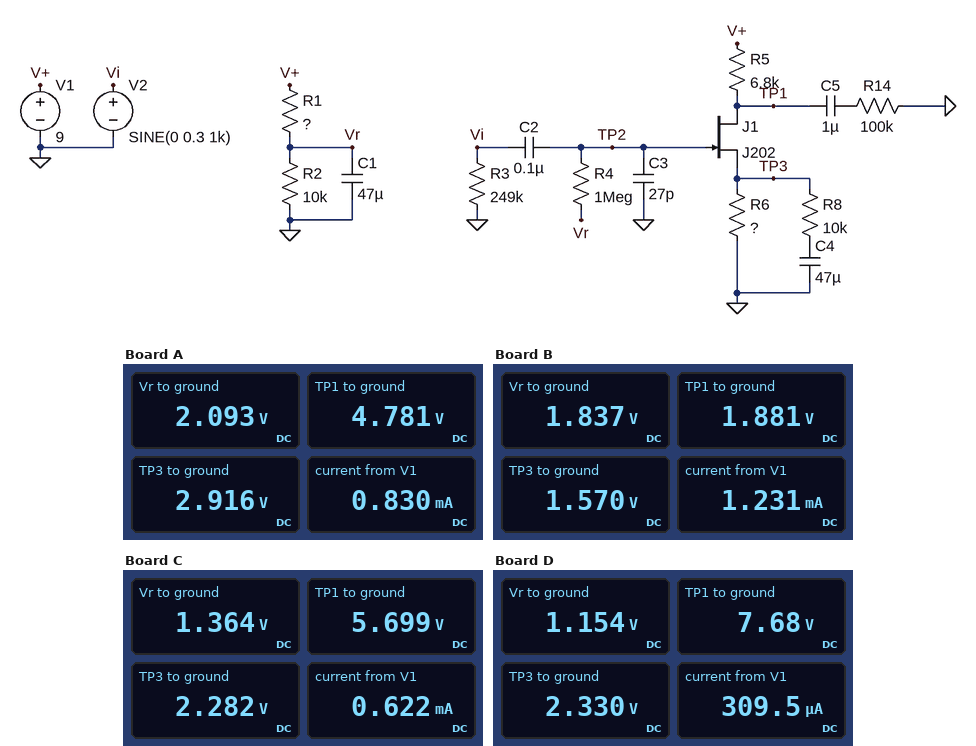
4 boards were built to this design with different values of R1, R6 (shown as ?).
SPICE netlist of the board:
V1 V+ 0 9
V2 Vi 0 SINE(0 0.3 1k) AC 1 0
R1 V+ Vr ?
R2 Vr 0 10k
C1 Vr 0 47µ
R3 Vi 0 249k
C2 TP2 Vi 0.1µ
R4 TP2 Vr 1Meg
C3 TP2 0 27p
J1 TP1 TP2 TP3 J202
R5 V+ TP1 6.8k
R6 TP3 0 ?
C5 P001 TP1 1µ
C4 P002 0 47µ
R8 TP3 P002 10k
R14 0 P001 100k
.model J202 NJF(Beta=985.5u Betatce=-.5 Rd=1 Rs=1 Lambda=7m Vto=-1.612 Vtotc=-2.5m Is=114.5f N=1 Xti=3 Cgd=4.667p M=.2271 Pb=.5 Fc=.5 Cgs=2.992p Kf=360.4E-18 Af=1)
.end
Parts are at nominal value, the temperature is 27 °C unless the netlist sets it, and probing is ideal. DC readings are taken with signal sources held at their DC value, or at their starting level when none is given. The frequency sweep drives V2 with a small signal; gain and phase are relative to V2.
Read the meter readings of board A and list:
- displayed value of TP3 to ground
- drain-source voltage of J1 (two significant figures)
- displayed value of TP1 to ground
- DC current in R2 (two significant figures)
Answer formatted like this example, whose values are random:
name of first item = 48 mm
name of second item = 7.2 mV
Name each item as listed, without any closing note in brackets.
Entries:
displayed value of TP3 to ground = 2.916 V
drain-source voltage of J1 = 1.9 V
displayed value of TP1 to ground = 4.781 V
DC current in R2 = 210 µA
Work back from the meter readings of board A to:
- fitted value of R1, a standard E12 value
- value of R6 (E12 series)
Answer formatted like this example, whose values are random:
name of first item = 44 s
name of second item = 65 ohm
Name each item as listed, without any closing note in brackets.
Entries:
fitted value of R1, a standard E12 value = 33 kΩ
value of R6 = 4.7 kΩ
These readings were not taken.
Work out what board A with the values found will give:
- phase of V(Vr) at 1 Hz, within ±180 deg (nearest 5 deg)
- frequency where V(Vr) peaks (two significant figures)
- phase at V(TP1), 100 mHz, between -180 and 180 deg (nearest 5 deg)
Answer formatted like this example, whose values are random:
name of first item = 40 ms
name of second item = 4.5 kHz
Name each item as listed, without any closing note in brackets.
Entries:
phase of V(Vr) at 1 Hz, within ±180 deg = -10 deg
frequency where V(Vr) peaks = 840 mHz
phase at V(TP1), 100 mHz, between -180 and 180 deg = -90 deg
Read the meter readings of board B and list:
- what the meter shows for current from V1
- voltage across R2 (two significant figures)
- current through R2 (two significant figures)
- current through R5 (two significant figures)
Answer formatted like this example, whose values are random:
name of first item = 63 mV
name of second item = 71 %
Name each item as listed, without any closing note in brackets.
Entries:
what the meter shows for current from V1 = 1.231 mA
voltage across R2 = 1.8 V
current through R2 = 180 µA
current through R5 = 1.0 mA
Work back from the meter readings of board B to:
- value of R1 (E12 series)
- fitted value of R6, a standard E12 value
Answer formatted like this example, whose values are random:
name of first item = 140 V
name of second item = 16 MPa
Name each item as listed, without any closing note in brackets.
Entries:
value of R1 = 39 kΩ
fitted value of R6, a standard E12 value = 1.5 kΩ
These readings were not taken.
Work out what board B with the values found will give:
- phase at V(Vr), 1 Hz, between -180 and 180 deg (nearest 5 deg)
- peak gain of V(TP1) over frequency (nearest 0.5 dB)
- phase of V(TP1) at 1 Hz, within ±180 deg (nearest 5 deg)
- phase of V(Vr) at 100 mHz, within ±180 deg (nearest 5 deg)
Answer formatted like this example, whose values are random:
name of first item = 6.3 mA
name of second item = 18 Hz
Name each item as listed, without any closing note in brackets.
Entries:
phase at V(Vr), 1 Hz, between -180 and 180 deg = -5 deg
peak gain of V(TP1) over frequency = -16.5 dB
phase of V(TP1) at 1 Hz, within ±180 deg = -120 deg
phase of V(Vr) at 100 mHz, within ±180 deg = 75 deg
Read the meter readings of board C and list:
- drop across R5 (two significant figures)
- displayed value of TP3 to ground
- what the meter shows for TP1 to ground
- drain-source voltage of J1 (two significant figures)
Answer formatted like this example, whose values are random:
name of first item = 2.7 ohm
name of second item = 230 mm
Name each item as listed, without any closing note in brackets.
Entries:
drop across R5 = 3.3 V
displayed value of TP3 to ground = 2.282 V
what the meter shows for TP1 to ground = 5.699 V
drain-source voltage of J1 = 3.4 V
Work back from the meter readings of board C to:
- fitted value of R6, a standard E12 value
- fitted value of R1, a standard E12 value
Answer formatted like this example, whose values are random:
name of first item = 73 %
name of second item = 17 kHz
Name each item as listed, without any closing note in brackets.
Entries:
fitted value of R6, a standard E12 value = 4.7 kΩ
fitted value of R1, a standard E12 value = 56 kΩ
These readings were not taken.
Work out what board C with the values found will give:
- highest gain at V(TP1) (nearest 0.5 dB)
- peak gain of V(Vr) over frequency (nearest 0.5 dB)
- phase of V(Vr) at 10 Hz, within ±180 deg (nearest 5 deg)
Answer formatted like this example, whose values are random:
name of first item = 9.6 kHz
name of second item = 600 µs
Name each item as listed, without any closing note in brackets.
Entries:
highest gain at V(TP1) = 4.0 dB
peak gain of V(Vr) over frequency = -55.5 dB
phase of V(Vr) at 10 Hz, within ±180 deg = -80 deg
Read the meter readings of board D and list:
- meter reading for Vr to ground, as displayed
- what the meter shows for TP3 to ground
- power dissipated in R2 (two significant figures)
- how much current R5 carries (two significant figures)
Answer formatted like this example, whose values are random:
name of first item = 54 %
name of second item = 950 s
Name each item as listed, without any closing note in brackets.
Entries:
meter reading for Vr to ground, as displayed = 1.154 V
what the meter shows for TP3 to ground = 2.330 V
power dissipated in R2 = 130 µW
how much current R5 carries = 190 µA
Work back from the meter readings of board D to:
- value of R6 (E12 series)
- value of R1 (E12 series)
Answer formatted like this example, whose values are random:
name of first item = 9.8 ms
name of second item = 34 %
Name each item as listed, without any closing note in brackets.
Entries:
value of R6 = 12 kΩ
value of R1 = 68 kΩ
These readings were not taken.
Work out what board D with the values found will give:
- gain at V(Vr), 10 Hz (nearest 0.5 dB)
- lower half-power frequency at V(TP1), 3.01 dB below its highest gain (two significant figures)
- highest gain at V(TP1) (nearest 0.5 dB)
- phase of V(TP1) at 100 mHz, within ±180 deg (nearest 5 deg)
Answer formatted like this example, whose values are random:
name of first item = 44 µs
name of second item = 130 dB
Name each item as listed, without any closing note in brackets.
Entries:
gain at V(Vr), 10 Hz = -69.5 dB
lower half-power frequency at V(TP1), 3.01 dB below its highest gain = 1.5 Hz
highest gain at V(TP1) = -0.5 dB
phase of V(TP1) at 100 mHz, within ±180 deg = -80 deg
